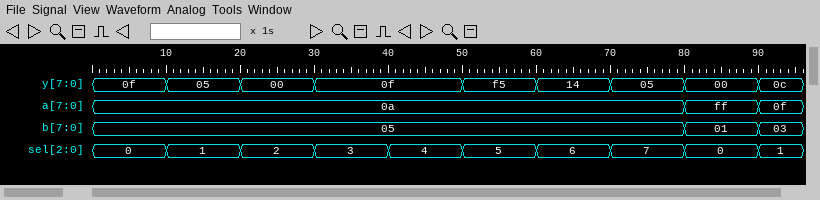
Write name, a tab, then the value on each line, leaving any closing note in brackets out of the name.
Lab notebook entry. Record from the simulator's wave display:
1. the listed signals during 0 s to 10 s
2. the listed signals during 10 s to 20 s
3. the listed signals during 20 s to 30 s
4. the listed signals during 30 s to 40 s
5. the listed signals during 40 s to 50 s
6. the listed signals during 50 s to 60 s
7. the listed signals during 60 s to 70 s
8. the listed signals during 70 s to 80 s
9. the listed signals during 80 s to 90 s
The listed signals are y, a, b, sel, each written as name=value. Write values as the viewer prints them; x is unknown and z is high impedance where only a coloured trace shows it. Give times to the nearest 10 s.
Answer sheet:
the listed signals during 0 s to 10 s	y=0f, a=0a, b=05, sel=0
the listed signals during 10 s to 20 s	y=05, a=0a, b=05, sel=1
the listed signals during 20 s to 30 s	y=00, a=0a, b=05, sel=2
the listed signals during 30 s to 40 s	y=0f, a=0a, b=05, sel=3
the listed signals during 40 s to 50 s	y=0f, a=0a, b=05, sel=4
the listed signals during 50 s to 60 s	y=f5, a=0a, b=05, sel=5
the listed signals during 60 s to 70 s	y=14, a=0a, b=05, sel=6
the listed signals during 70 s to 80 s	y=05, a=0a, b=05, sel=7
the listed signals during 80 s to 90 s	y=00, a=ff, b=01, sel=0
